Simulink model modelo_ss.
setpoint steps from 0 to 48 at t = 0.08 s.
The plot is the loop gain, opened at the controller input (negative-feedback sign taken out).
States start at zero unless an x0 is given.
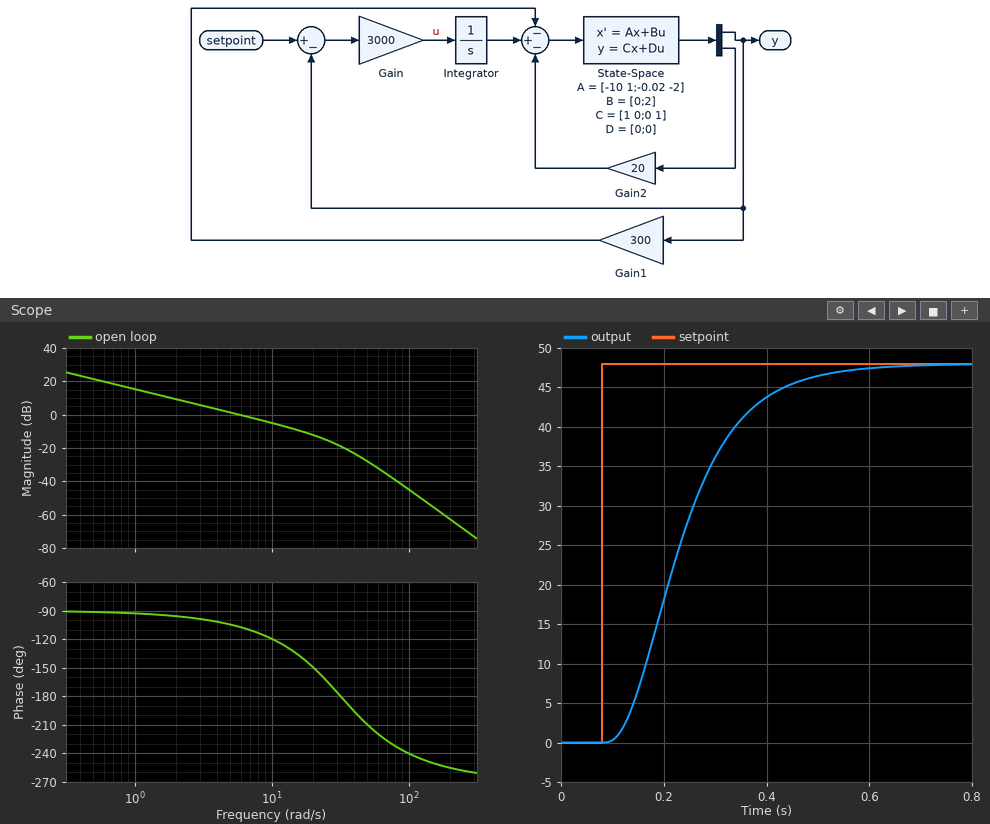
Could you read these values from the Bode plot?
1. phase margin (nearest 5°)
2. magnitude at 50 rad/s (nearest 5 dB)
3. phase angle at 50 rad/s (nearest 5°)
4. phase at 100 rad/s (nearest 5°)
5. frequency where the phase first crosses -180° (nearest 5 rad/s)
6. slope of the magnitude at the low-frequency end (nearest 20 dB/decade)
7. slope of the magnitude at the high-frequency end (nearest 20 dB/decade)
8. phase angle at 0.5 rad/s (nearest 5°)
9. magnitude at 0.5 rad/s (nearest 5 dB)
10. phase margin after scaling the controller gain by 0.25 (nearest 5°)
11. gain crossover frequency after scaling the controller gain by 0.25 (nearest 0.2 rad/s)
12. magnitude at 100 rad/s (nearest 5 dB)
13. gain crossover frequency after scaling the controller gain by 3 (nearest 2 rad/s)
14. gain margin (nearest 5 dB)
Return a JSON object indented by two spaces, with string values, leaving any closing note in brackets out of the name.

{
  "phase margin": "75°",
  "magnitude at 50 rad/s": "-30 dB",
  "phase angle at 50 rad/s": "-210°",
  "phase at 100 rad/s": "-240°",
  "frequency where the phase first crosses -180°": "30 rad/s",
  "slope of the magnitude at the low-frequency end": "-20 dB/decade",
  "slope of the magnitude at the high-frequency end": "-60 dB/decade",
  "phase angle at 0.5 rad/s": "-90°",
  "magnitude at 0.5 rad/s": "20 dB",
  "phase margin after scaling the controller gain by 0.25": "85°",
  "gain crossover frequency after scaling the controller gain by 0.25": "1.4 rad/s",
  "magnitude at 100 rad/s": "-45 dB",
  "gain crossover frequency after scaling the controller gain by 3": "16 rad/s",
  "gain margin": "20 dB"
}
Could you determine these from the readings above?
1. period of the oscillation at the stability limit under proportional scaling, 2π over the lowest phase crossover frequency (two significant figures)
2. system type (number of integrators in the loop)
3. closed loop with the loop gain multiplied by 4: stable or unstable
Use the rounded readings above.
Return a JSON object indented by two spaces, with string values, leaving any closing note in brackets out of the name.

{
  "period of the oscillation at the stability limit under proportional scaling, 2π over the lowest phase crossover frequency": "0.21 s",
  "system type": "1",
  "closed loop with the loop gain multiplied by 4: stable or unstable": "stable"
}
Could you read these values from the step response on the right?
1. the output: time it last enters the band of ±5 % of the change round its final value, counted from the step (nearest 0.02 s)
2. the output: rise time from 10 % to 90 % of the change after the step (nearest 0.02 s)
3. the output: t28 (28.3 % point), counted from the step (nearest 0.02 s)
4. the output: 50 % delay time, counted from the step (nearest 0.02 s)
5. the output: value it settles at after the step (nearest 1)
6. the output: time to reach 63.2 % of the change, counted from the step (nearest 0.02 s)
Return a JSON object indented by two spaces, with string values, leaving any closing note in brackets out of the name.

{
  "the output: time it last enters the band of ±5 % of the change round its final value, counted from the step": "0.38 s",
  "the output: rise time from 10 % to 90 % of the change after the step": "0.24 s",
  "the output: t28 (28.3 % point), counted from the step": "0.10 s",
  "the output: 50 % delay time, counted from the step": "0.14 s",
  "the output: value it settles at after the step": "48",
  "the output: time to reach 63.2 % of the change, counted from the step": "0.18 s"
}
